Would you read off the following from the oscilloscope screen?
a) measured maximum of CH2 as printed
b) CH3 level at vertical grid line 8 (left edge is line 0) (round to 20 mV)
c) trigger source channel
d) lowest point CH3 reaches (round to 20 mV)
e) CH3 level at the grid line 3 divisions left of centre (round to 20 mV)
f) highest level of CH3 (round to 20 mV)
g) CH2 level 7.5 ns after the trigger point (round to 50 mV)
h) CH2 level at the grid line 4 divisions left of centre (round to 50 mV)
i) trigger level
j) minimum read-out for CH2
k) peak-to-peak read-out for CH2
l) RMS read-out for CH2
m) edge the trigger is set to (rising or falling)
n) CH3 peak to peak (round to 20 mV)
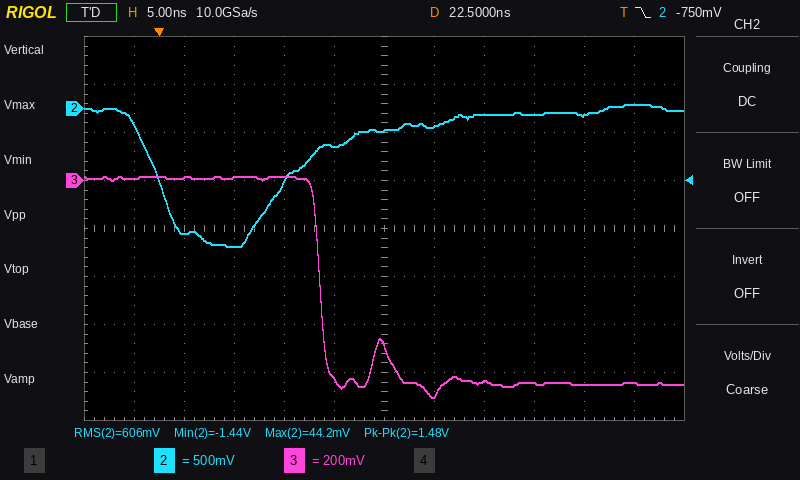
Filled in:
44.2 mV
-840 mV
CH2
-900 mV
20 mV
20 mV
-1.45 V
-1.30 V
-750 mV
-1.44 V
1.48 V
606 mV
falling
920 mV
